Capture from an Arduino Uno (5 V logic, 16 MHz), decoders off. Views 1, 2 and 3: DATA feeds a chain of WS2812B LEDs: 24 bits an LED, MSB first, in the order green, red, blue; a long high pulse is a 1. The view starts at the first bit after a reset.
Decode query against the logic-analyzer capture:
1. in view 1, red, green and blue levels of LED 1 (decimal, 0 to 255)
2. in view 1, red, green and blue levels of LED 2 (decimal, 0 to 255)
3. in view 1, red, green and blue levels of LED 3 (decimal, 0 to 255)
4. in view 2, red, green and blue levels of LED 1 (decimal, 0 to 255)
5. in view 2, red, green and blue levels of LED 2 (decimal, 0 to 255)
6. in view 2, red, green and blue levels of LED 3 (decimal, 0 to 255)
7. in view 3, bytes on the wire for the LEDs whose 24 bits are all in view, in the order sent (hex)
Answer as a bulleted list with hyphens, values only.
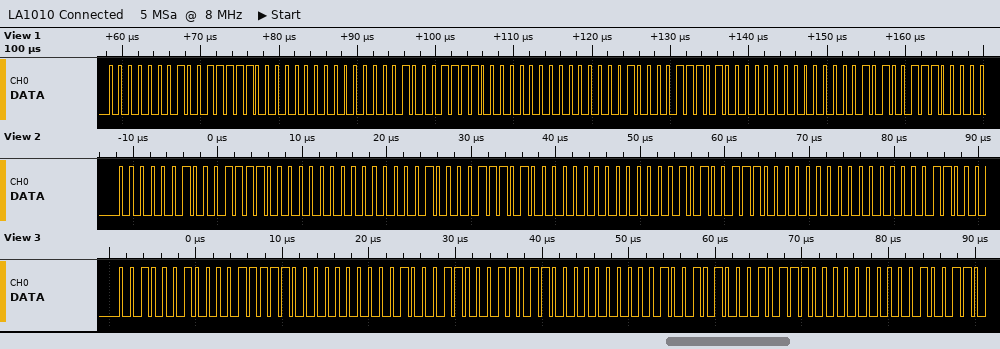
- 62, 1, 0
- 60, 2, 0
- 58, 4, 0
- 60, 2, 0
- 58, 4, 0
- 56, 5, 0
- 22 1F 00 23 1B 00 25 17 00
